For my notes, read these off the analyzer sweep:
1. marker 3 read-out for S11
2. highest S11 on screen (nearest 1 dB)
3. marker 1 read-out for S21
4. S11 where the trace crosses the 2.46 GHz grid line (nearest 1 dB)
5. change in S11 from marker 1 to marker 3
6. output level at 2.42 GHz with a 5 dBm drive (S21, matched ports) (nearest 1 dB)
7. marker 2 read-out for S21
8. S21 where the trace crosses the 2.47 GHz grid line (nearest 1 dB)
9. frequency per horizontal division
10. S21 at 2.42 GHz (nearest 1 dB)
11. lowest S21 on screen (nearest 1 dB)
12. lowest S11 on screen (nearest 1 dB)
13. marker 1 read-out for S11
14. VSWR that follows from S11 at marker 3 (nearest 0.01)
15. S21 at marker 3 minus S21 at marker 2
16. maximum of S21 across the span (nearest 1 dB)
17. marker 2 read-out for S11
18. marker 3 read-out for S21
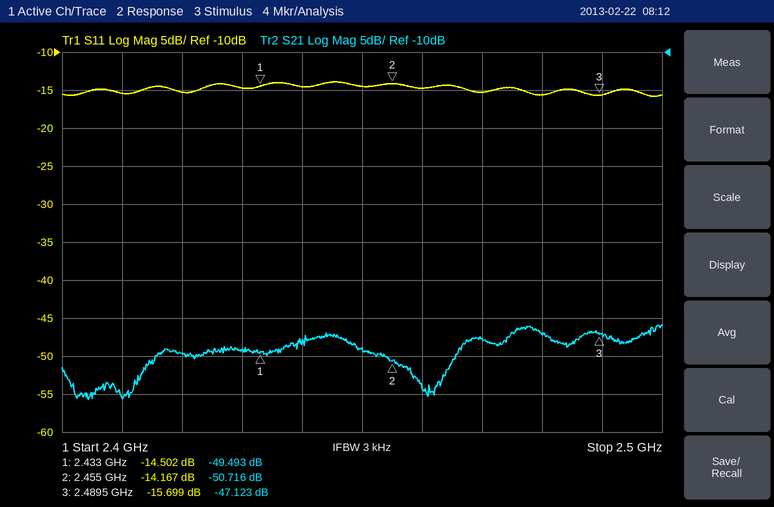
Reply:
-15.699 dB
-14 dB
-49.493 dB
-15 dB
-1.197 dB
-45 dBm
-50.716 dB
-48 dB
10 MHz
-50 dB
-56 dB
-16 dB
-14.502 dB
1.39
3.593 dB
-46 dB
-14.167 dB
-47.123 dB
